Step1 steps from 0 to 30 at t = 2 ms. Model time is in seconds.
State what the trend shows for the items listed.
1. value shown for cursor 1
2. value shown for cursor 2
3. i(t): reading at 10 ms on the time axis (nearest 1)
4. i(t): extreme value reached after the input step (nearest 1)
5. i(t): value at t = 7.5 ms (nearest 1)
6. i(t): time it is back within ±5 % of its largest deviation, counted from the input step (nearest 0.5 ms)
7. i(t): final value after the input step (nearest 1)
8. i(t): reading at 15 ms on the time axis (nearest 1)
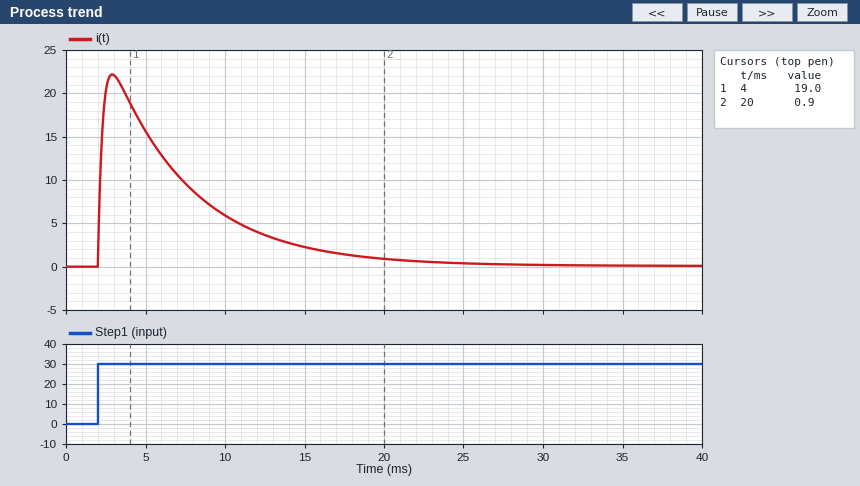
19.0
0.9
6
22
10
16.5 ms
0
2
